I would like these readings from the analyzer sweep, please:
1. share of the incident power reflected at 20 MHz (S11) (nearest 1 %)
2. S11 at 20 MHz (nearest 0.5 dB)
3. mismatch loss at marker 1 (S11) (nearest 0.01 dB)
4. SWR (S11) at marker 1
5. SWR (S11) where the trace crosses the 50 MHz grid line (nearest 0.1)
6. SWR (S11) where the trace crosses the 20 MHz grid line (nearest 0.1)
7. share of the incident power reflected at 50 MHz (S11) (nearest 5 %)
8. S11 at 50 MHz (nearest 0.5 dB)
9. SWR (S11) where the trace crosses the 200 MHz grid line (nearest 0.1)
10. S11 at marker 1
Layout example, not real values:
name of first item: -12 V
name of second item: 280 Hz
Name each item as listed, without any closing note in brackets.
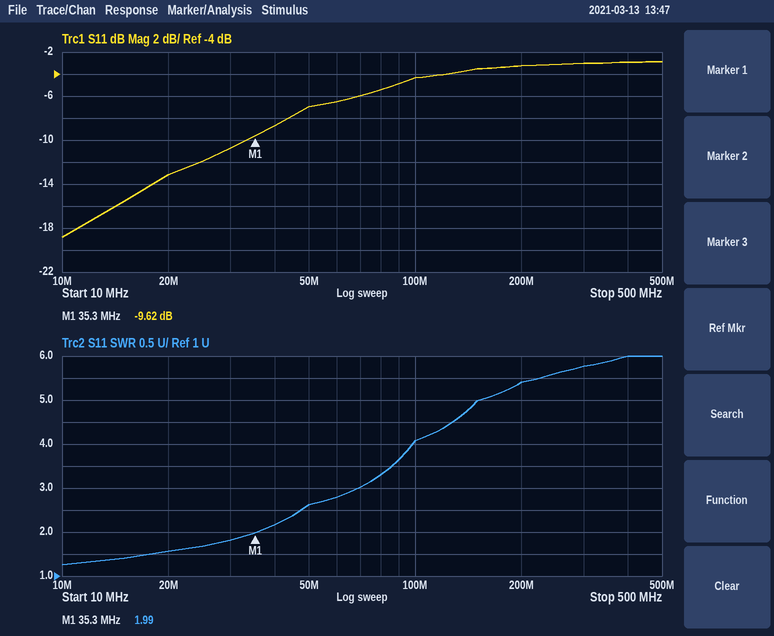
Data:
share of the incident power reflected at 20 MHz (S11): 5 %
S11 at 20 MHz: -13.0 dB
mismatch loss at marker 1 (S11): 0.50 dB
SWR (S11) at marker 1: 1.99
SWR (S11) where the trace crosses the 50 MHz grid line: 2.6
SWR (S11) where the trace crosses the 20 MHz grid line: 1.6
share of the incident power reflected at 50 MHz (S11): 20 %
S11 at 50 MHz: -7.0 dB
SWR (S11) where the trace crosses the 200 MHz grid line: 5.4
S11 at marker 1: -9.62 dB
